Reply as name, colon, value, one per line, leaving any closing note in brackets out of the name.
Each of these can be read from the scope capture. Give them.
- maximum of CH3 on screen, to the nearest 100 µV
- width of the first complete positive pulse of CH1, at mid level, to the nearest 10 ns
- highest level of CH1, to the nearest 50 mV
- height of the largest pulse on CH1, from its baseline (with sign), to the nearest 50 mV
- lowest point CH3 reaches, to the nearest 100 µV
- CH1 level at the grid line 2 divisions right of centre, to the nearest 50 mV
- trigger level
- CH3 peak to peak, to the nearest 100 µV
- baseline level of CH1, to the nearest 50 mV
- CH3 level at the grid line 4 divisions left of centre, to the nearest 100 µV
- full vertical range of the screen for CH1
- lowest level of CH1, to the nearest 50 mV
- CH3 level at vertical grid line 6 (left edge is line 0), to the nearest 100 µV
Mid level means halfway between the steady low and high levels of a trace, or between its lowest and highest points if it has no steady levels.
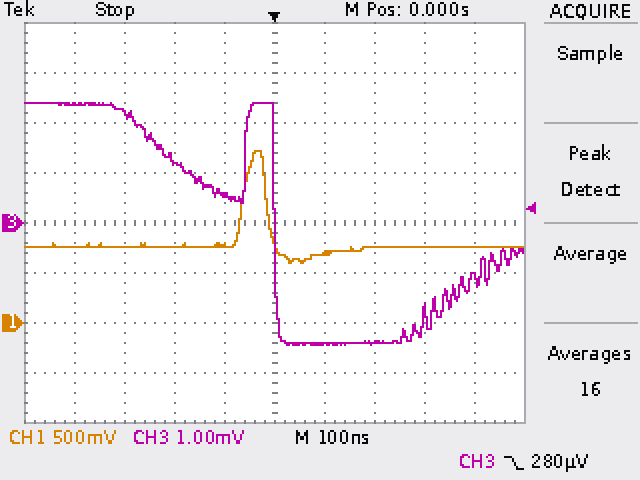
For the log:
maximum of CH3 on screen, to the nearest 100 µV: 2.4 mV
width of the first complete positive pulse of CH1, at mid level, to the nearest 10 ns: 50 ns
highest level of CH1, to the nearest 50 mV: 1.70 V
height of the largest pulse on CH1, from its baseline (with sign), to the nearest 50 mV: +950 mV
lowest point CH3 reaches, to the nearest 100 µV: -2.4 mV
CH1 level at the grid line 2 divisions right of centre, to the nearest 50 mV: 750 mV
trigger level: 280 µV
CH3 peak to peak, to the nearest 100 µV: 4.8 mV
baseline level of CH1, to the nearest 50 mV: 750 mV
CH3 level at the grid line 4 divisions left of centre, to the nearest 100 µV: 2.4 mV
full vertical range of the screen for CH1: 4 V
lowest level of CH1, to the nearest 50 mV: 600 mV
CH3 level at vertical grid line 6 (left edge is line 0), to the nearest 100 µV: -2.4 mV
